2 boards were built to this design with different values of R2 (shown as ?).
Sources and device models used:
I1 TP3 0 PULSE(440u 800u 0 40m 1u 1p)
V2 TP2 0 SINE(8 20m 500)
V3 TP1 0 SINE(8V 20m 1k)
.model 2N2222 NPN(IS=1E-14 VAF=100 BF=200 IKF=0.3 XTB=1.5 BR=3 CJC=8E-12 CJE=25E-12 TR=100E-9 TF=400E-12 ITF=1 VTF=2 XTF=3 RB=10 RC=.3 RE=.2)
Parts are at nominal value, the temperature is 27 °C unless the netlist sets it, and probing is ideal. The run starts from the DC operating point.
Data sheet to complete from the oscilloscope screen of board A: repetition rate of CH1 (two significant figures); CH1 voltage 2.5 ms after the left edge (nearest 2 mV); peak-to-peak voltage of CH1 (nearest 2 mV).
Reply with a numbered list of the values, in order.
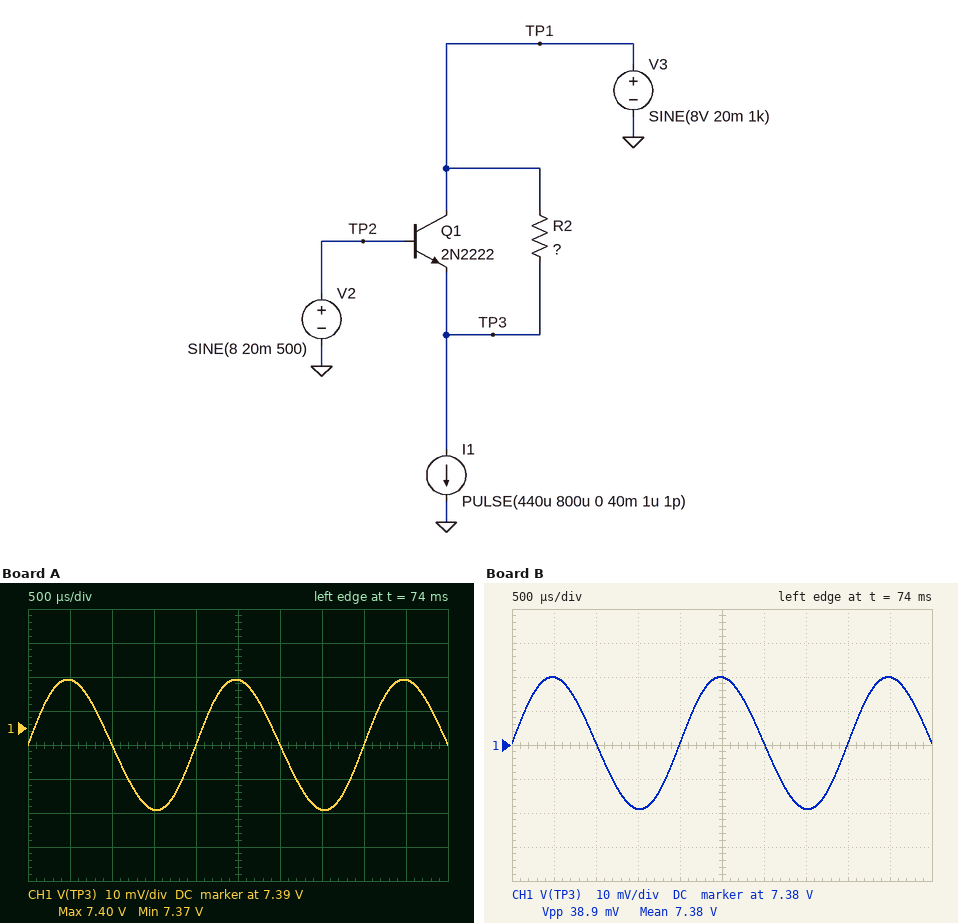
1. 500 Hz
2. 7.404 V
3. 38 mV
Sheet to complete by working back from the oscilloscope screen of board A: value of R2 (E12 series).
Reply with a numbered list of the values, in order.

1. 2.7 kΩ
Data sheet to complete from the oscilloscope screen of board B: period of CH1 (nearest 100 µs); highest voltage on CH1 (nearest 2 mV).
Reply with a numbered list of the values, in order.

1. 2.0 ms
2. 7.400 V
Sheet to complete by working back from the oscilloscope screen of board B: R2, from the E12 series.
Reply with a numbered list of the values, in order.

1. 3.3 kΩ
